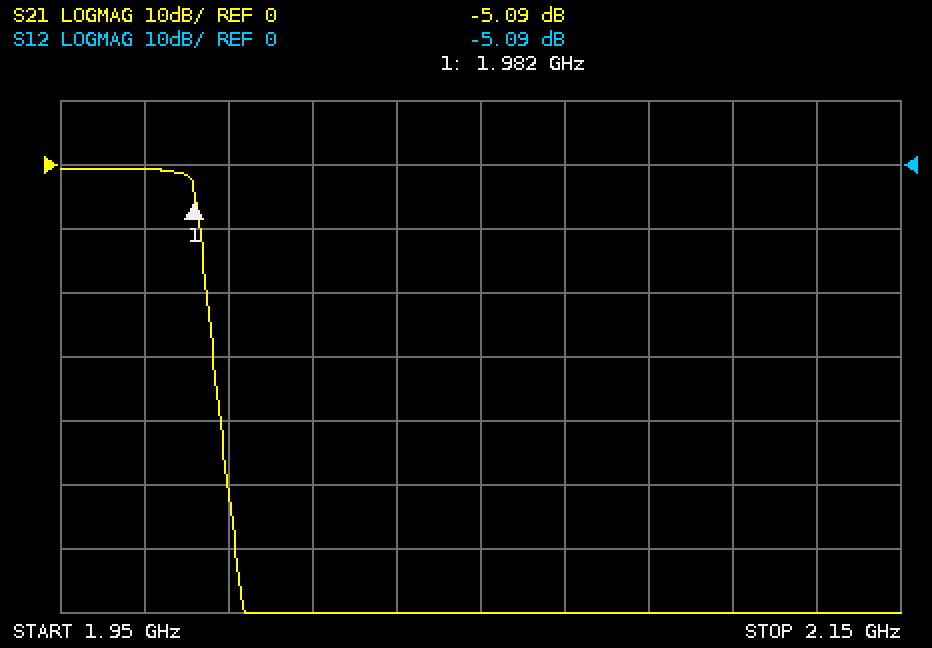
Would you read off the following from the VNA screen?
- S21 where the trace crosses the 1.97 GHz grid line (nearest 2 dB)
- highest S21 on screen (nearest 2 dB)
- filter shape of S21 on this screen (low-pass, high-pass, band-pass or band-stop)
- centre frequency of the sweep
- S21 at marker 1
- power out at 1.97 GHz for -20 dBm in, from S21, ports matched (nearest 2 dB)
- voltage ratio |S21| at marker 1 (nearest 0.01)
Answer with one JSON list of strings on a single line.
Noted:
["0 dB", "0 dB", "low-pass", "2.05 GHz", "-5.09 dB", "-20 dBm", "0.56"]
